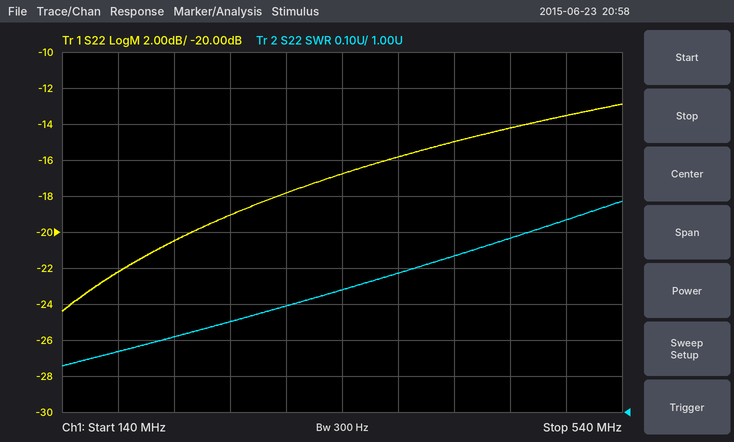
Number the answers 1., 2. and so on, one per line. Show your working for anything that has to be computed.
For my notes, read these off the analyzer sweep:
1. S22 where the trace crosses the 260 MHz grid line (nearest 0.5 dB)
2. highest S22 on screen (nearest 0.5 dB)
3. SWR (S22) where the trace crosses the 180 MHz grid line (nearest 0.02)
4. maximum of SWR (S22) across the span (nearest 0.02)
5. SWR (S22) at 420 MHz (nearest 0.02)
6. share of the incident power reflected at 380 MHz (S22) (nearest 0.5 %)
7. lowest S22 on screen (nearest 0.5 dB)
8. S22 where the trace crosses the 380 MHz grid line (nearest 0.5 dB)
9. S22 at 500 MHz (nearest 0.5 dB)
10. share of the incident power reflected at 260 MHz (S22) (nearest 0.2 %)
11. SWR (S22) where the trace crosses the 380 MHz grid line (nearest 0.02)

1. -19.0 dB
2. -13.0 dB
3. 1.16
4. 1.58
5. 1.44
6. 10^(-16/10) ≈ 2.5 %
7. -24.5 dB
8. -16.0 dB
9. -13.5 dB
10. 10^(-19/10) ≈ 1.26 %, so 1.2 % to the nearest 0.2 %
11. 1.38
